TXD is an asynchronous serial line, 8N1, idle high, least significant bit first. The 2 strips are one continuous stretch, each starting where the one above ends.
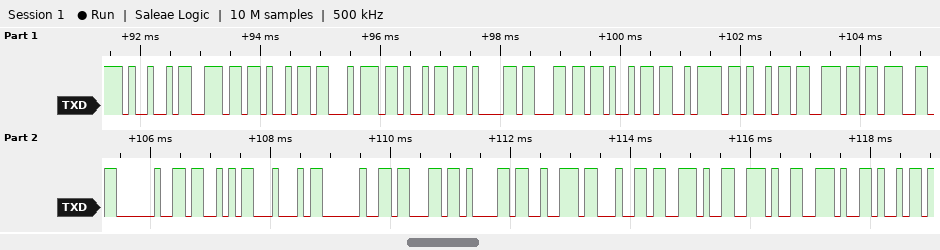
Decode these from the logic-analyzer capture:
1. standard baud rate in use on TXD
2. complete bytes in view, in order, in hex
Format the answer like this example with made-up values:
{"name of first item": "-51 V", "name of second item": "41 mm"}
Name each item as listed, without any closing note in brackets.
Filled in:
{"standard baud rate in use on TXD": "9600 baud", "complete bytes in view, in order, in hex": "49 6E 69 74 69 61 6C 69 7A 69 6E 67 20 53 44 20 63 61 72 64 2E 2E 2E 69"}
